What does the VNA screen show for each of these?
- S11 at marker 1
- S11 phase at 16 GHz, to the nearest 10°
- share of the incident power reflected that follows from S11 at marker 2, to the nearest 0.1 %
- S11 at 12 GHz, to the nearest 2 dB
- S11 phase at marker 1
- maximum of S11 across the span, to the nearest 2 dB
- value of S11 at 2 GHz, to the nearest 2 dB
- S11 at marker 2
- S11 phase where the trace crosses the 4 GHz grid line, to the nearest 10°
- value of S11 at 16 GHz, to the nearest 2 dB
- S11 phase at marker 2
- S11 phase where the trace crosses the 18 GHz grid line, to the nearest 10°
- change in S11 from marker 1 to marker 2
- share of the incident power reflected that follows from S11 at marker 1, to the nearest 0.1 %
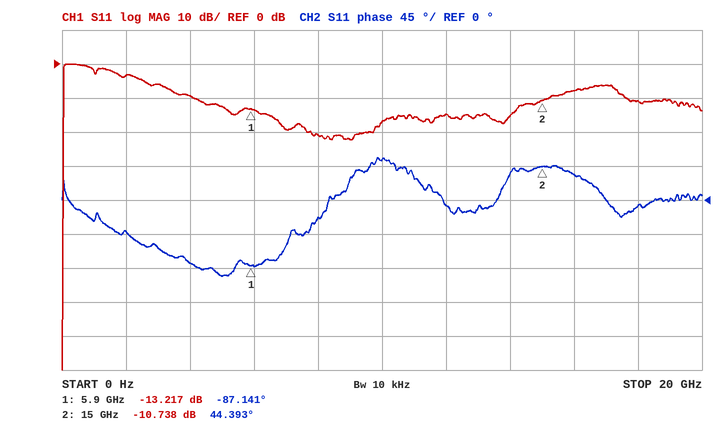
-13.217 dB
30°
8.4 %
-14 dB
-87.141°
0 dB
-4 dB
-10.738 dB
-80°
-8 dB
44.393°
-10°
2.479 dB
4.8 %
